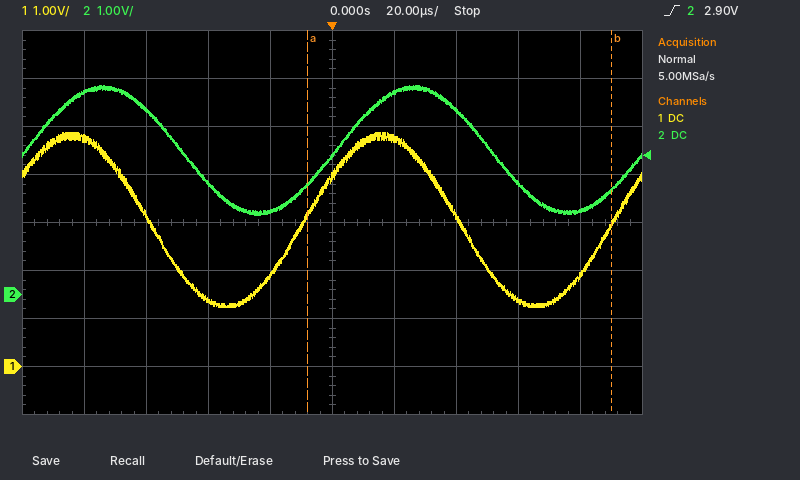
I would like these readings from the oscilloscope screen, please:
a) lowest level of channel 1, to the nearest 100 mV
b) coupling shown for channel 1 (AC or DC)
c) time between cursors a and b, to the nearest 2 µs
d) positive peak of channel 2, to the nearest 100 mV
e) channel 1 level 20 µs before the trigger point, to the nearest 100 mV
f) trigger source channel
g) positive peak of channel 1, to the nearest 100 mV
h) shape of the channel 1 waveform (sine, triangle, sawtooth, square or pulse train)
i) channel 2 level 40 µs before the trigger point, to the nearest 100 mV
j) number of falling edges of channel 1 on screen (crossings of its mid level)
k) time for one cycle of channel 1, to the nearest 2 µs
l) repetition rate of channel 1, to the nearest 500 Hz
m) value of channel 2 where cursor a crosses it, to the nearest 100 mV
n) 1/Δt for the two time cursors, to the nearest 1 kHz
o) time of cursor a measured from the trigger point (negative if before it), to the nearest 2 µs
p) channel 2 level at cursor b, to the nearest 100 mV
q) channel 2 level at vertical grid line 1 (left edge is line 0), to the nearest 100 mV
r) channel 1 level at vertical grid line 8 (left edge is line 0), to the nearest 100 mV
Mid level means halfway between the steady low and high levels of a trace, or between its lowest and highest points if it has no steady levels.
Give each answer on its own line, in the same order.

1.2 V
DC
98 µs
4.4 V
1.9 V
channel 2
4.9 V
sine
2.3 V
2
100 µs
10.0 kHz
2.3 V
10 kHz
-8 µs
2.2 V
4.2 V
1.4 V
